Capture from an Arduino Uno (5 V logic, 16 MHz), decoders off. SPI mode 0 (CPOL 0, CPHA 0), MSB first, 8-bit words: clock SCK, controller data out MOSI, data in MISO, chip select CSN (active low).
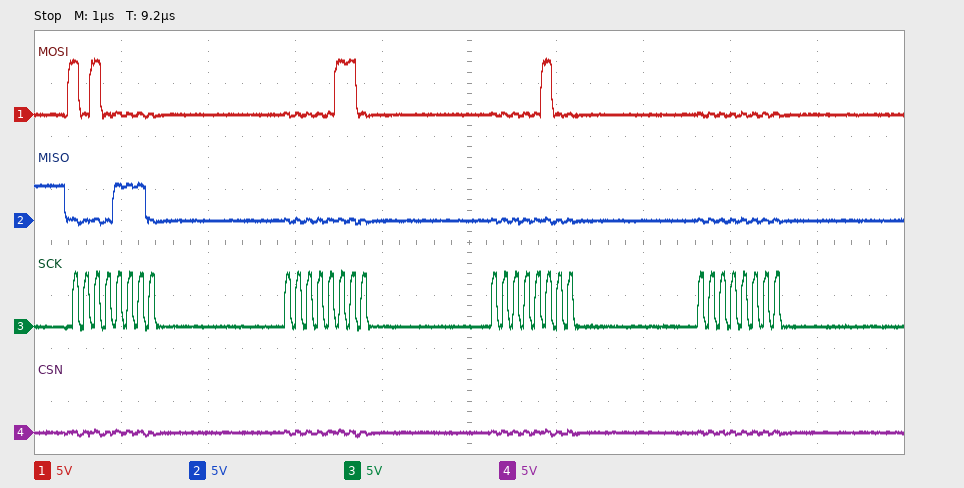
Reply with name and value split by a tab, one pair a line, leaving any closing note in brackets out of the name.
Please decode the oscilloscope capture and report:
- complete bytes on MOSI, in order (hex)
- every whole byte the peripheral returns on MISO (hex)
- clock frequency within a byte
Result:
complete bytes on MOSI, in order	A0 06 04 00
every whole byte the peripheral returns on MISO	0E 00 00 00
clock frequency within a byte	8 MHz
